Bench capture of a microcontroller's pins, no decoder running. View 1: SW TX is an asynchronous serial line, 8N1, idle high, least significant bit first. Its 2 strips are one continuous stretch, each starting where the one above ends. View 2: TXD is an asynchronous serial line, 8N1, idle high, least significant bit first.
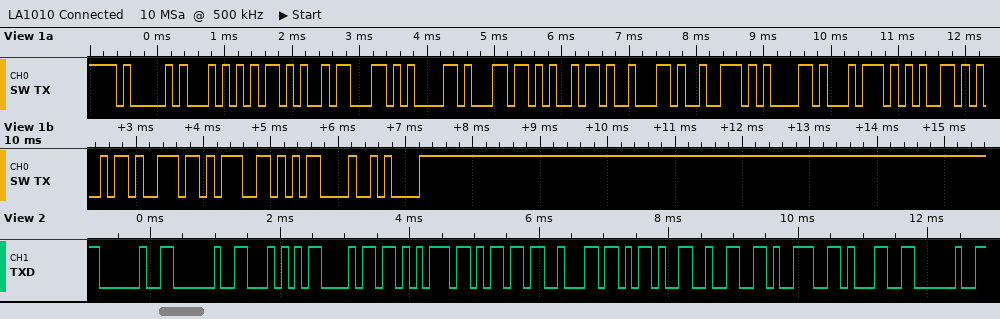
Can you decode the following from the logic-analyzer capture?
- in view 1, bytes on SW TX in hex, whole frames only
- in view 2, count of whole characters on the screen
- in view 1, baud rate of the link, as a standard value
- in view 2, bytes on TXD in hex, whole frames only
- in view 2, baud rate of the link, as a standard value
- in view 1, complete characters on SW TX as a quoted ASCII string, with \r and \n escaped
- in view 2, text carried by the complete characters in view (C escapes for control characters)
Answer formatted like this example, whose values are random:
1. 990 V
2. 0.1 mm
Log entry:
1. 41 54 2B 63 61 6C 69 62 72 61 74 65 69 6E 67 0D 0A
2. 12
3. 9600 baud
4. 20 20 54 68 75 6D 62 2D 32 39 31 20
5. 9600 baud
6. "AT+calibrateing\r\n"
7. "  Thumb-291 "
